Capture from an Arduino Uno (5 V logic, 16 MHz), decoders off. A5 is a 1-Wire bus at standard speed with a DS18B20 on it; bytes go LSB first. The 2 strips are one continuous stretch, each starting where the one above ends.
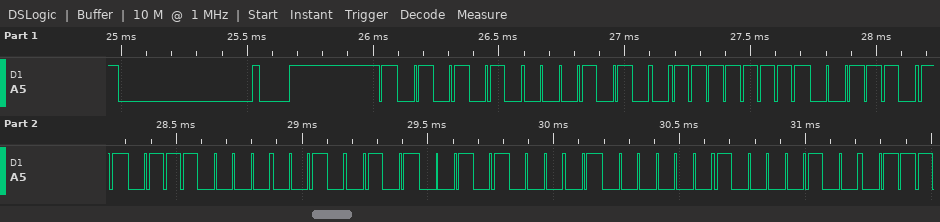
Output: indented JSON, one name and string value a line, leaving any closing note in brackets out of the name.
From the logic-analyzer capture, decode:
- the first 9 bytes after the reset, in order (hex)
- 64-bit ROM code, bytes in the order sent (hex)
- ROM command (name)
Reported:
{
  "the first 9 bytes after the reset, in order": "55 28 FF DC 0E A4 14 02 21",
  "64-bit ROM code, bytes in the order sent": "28 FF DC 0E A4 14 02 21",
  "ROM command": "Match ROM"
}
